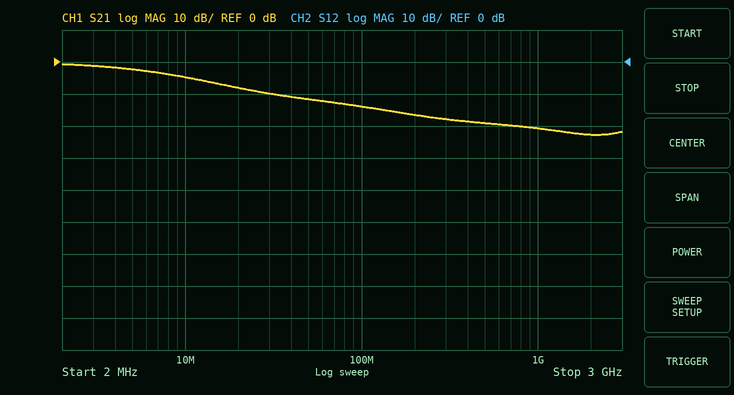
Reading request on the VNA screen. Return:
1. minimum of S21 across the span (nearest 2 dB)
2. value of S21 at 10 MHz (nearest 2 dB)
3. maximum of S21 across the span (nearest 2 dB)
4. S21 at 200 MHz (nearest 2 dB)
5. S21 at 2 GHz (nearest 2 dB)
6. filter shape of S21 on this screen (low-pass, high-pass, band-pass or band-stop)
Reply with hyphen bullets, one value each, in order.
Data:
- -22 dB
- -4 dB
- 0 dB
- -16 dB
- -22 dB
- low-pass
